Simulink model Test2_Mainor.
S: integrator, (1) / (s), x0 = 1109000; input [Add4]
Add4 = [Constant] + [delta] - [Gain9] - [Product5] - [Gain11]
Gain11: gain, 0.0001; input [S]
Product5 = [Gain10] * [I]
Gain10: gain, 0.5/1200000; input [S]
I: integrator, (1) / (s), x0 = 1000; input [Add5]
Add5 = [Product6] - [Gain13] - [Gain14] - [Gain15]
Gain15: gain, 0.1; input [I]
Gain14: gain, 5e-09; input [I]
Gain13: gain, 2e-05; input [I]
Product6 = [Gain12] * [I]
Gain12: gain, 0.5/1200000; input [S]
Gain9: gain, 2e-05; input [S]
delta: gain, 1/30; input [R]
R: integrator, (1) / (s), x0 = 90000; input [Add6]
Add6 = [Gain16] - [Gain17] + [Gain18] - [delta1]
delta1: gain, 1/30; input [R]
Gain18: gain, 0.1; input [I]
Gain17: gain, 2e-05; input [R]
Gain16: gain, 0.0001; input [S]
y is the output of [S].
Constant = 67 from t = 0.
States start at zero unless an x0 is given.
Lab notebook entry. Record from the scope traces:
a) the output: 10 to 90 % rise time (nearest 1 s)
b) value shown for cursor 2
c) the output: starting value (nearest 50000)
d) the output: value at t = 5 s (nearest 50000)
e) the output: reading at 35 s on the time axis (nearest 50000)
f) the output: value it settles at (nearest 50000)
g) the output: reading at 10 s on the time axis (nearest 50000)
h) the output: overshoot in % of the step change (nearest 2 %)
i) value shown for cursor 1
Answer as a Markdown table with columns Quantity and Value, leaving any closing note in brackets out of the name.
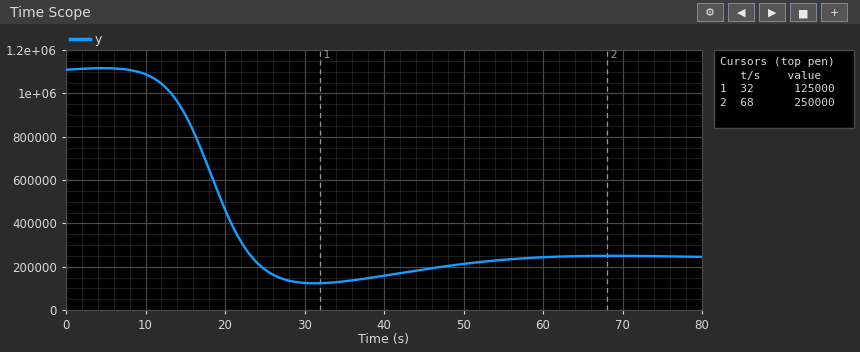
| Quantity | Value |
|---|---|
| the output: 10 to 90 % rise time | 9 s |
| value shown for cursor 2 | 250000 |
| the output: starting value | 1100000 |
| the output: value at t = 5 s | 1100000 |
| the output: reading at 35 s on the time axis | 150000 |
| the output: value it settles at | 250000 |
| the output: reading at 10 s on the time axis | 1100000 |
| the output: overshoot in % of the step change | 14 % |
| value shown for cursor 1 | 125000 |
